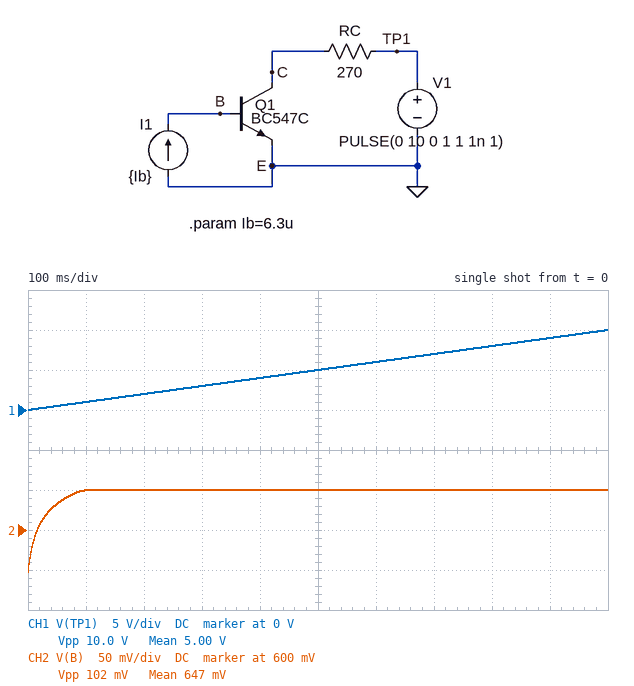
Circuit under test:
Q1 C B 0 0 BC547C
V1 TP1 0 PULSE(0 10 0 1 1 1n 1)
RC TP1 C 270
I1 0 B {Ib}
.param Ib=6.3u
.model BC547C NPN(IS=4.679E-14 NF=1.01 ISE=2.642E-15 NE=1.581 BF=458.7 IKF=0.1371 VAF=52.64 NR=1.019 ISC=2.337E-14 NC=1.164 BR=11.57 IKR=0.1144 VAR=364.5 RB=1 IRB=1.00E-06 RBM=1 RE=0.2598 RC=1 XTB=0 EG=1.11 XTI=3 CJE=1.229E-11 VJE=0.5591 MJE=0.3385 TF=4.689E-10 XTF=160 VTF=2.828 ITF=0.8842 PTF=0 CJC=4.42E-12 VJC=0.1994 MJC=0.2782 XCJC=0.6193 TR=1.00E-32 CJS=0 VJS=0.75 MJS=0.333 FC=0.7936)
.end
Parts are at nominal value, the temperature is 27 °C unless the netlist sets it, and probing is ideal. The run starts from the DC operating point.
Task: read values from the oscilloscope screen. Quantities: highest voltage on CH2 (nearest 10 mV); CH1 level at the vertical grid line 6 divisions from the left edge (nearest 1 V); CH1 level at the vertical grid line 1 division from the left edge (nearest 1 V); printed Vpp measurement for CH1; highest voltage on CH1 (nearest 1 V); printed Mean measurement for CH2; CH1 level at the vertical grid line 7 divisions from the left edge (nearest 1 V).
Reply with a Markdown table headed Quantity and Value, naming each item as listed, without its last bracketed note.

| Quantity | Value |
|---|---|
| highest voltage on CH2 | 650 mV |
| CH1 level at the vertical grid line 6 divisions from the left edge | 6 V |
| CH1 level at the vertical grid line 1 division from the left edge | 1 V |
| printed Vpp measurement for CH1 | 10.0 V |
| highest voltage on CH1 | 10 V |
| printed Mean measurement for CH2 | 647 mV |
| CH1 level at the vertical grid line 7 divisions from the left edge | 7 V |
